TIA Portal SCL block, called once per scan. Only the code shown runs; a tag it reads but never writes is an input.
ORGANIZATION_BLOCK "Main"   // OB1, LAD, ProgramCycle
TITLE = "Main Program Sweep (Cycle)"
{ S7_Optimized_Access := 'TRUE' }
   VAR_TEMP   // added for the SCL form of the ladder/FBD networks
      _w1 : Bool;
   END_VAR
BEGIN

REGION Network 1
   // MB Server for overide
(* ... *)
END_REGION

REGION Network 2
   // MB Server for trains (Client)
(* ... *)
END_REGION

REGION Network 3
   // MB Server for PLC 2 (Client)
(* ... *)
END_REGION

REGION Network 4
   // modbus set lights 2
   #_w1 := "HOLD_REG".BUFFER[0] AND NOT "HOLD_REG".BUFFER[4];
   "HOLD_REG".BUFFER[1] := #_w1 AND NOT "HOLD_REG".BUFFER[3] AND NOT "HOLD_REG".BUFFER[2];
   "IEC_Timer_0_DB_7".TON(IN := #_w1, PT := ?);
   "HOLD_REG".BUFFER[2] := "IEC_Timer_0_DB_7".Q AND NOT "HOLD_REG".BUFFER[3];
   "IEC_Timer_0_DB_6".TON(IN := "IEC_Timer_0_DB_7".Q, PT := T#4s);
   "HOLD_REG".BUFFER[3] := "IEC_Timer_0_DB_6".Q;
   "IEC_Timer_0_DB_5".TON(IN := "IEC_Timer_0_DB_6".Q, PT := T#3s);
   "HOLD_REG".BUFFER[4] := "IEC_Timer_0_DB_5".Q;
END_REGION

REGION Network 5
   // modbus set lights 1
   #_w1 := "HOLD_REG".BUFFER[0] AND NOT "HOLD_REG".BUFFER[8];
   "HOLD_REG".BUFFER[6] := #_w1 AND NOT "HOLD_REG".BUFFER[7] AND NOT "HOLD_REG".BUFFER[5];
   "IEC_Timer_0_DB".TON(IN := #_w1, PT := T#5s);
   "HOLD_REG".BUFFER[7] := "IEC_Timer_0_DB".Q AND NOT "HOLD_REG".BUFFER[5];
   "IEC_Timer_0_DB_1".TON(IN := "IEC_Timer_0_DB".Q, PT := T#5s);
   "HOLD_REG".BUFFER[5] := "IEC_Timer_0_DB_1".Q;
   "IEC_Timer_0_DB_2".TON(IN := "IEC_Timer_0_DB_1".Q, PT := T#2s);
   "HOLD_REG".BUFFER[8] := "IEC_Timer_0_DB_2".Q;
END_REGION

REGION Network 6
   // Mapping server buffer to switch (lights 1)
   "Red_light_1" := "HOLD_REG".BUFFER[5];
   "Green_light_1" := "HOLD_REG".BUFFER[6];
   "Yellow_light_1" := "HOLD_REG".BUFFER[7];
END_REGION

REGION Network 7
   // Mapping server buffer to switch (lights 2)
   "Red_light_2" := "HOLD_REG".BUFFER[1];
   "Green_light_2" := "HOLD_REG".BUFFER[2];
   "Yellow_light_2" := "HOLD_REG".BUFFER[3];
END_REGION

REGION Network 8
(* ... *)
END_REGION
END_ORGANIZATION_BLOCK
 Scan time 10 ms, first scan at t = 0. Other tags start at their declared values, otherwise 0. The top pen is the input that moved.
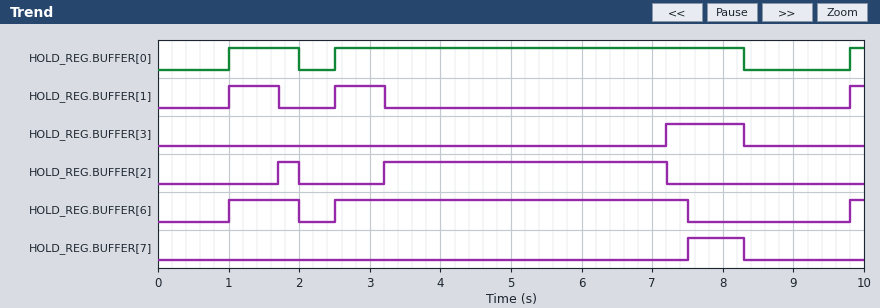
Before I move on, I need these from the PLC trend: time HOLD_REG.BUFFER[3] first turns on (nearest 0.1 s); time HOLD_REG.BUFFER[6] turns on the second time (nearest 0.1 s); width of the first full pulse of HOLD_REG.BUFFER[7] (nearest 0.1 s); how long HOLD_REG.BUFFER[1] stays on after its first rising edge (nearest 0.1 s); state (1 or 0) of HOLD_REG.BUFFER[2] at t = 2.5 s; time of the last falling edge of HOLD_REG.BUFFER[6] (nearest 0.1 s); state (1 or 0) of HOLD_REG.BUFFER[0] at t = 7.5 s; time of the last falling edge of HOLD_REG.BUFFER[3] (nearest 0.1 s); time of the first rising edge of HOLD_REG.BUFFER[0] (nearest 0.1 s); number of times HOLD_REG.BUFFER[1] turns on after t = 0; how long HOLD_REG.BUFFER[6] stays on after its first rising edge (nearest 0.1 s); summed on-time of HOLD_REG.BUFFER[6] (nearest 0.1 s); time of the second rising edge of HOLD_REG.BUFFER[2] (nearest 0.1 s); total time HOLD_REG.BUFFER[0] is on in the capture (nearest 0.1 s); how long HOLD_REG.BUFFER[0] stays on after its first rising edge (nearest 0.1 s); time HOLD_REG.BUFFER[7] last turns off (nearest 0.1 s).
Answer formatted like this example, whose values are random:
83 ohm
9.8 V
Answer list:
7.2 s
2.5 s
0.8 s
0.7 s
0
7.5 s
1
8.3 s
1.0 s
3
1.0 s
6.2 s
3.2 s
7.0 s
1.0 s
8.3 s
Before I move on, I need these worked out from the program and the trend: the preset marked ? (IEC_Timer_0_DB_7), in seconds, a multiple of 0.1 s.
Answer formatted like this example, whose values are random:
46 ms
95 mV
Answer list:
0.7 s
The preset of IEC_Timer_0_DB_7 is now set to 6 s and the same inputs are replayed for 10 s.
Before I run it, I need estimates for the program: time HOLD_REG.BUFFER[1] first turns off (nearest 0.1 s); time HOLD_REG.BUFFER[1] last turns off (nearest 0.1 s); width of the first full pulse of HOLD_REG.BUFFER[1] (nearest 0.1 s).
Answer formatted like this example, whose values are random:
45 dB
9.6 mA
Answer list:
2.0 s
8.3 s
1.0 s
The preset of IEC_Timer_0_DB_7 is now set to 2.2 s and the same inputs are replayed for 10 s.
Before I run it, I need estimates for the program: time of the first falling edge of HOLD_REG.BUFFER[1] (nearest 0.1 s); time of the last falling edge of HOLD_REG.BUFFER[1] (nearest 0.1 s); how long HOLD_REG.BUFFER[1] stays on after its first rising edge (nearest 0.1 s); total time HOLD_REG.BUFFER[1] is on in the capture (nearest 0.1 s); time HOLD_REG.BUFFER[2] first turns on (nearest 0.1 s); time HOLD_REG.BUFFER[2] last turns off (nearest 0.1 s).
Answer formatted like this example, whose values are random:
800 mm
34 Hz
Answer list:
2.0 s
4.7 s
1.0 s
3.4 s
4.7 s
8.3 s
